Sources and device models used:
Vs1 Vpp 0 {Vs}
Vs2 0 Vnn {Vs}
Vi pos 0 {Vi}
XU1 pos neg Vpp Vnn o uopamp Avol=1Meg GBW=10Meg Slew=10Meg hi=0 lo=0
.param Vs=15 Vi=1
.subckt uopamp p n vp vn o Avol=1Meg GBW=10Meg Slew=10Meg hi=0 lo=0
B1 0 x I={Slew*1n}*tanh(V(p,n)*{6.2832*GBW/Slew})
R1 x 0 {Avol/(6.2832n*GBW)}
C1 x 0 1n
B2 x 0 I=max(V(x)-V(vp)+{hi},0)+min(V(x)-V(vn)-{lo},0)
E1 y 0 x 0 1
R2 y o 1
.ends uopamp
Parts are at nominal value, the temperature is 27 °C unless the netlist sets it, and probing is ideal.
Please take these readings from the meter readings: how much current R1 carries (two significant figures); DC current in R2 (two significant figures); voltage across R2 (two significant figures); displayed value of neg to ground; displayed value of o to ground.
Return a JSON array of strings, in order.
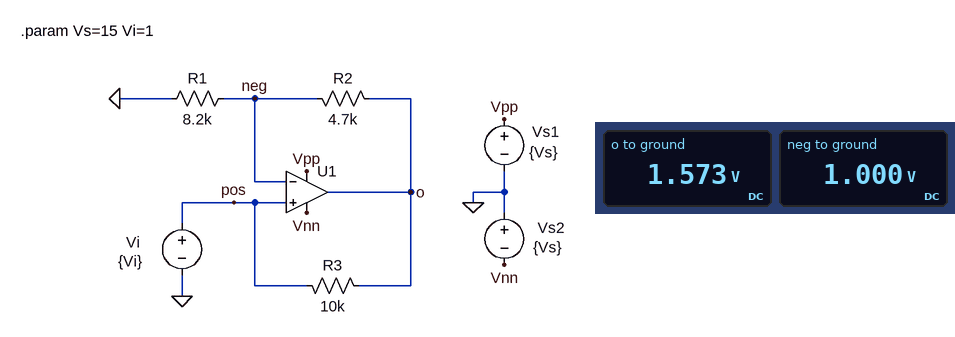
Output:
["120 µA", "120 µA", "570 mV", "1.000 V", "1.573 V"]
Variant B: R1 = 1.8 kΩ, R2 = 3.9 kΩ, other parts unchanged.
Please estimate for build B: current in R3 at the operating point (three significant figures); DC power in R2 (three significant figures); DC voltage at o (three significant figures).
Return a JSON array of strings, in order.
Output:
["217 µA", "1.20 mW", "3.17 V"]
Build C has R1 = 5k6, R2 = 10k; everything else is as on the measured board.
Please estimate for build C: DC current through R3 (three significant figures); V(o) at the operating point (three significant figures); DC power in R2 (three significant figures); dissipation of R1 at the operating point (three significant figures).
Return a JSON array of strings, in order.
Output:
["179 µA", "2.79 V", "319 µW", "179 µW"]
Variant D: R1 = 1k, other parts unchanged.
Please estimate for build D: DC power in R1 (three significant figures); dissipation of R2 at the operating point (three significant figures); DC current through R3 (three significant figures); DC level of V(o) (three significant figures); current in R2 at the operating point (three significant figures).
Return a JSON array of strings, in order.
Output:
["1.00 mW", "4.70 mW", "470 µA", "5.70 V", "1.00 mA"]
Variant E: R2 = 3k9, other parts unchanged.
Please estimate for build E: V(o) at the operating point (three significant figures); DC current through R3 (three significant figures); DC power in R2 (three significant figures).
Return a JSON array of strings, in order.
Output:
["1.48 V", "47.6 µA", "58.0 µW"]
